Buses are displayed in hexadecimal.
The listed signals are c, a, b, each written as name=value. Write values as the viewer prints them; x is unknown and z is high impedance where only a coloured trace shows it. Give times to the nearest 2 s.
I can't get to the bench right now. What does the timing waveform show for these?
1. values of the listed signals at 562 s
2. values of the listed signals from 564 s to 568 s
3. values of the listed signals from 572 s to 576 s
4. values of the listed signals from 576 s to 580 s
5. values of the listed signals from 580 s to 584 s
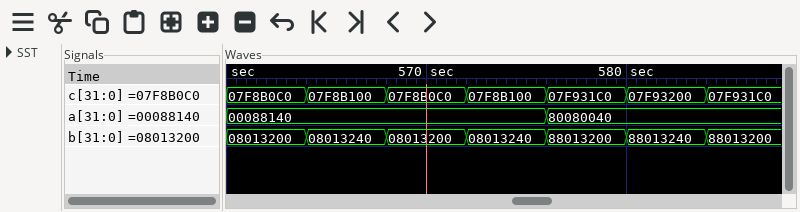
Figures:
c=07F8B0C0, a=00088140, b=08013200
c=07F8B100, a=00088140, b=08013240
c=07F8B100, a=00088140, b=08013240
c=07F931C0, a=80080040, b=88013200
c=07F93200, a=80080040, b=88013240
